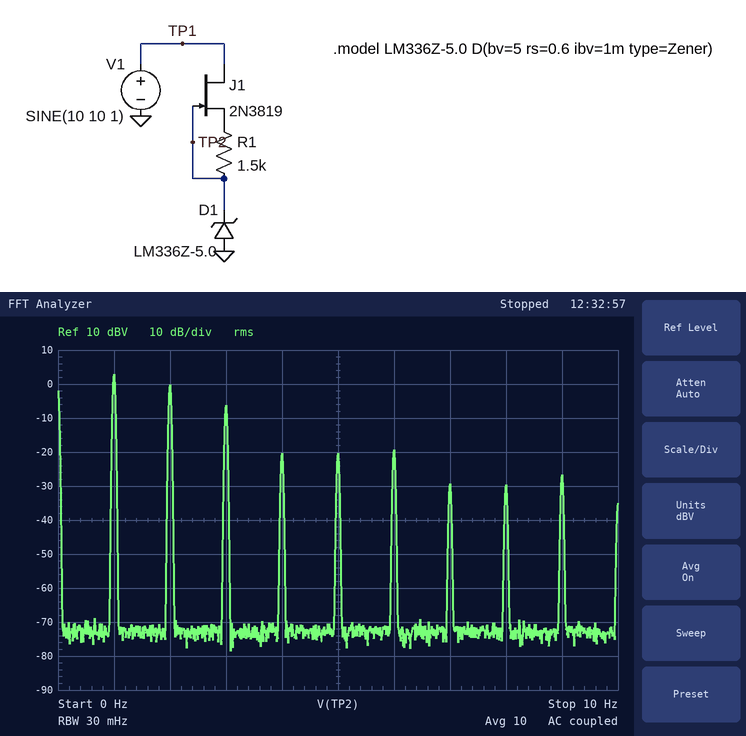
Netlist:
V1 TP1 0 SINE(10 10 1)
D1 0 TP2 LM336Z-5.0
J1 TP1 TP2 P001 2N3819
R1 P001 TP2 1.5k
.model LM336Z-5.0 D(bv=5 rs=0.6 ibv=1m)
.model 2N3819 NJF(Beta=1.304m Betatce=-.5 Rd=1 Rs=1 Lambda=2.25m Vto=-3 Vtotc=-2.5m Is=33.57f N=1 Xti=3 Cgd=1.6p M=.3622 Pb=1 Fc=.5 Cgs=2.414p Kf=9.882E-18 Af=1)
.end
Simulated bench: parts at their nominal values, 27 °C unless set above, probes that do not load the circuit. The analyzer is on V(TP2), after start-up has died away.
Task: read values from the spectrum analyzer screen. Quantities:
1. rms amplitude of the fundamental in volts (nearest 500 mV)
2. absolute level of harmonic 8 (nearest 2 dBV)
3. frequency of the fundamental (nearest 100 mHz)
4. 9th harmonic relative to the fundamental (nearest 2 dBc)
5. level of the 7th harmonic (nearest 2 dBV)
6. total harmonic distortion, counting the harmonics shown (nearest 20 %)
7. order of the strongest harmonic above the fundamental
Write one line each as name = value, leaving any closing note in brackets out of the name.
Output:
rms amplitude of the fundamental in volts = 1.5 V
absolute level of harmonic 8 = -30 dBV
frequency of the fundamental = 1.0 Hz
9th harmonic relative to the fundamental = -30 dBc
level of the 7th harmonic = -30 dBV
total harmonic distortion, counting the harmonics shown = 80 %
order of the strongest harmonic above the fundamental = 2
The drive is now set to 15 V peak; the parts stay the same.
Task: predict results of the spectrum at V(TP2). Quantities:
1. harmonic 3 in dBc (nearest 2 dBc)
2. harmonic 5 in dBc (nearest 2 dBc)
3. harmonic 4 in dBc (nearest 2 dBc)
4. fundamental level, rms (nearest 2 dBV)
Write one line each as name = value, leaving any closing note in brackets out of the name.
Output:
harmonic 3 in dBc = -20 dBc
harmonic 5 in dBc = -18 dBc
harmonic 4 in dBc = -18 dBc
fundamental level, rms = 8 dBV
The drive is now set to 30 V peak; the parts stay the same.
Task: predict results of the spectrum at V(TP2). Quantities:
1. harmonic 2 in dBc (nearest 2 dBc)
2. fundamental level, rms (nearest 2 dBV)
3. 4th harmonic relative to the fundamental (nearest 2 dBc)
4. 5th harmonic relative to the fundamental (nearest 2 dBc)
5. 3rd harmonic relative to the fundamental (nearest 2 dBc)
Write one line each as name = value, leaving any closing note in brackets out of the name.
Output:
harmonic 2 in dBc = -8 dBc
fundamental level, rms = 14 dBV
4th harmonic relative to the fundamental = -18 dBc
5th harmonic relative to the fundamental = -36 dBc
3rd harmonic relative to the fundamental = -34 dBc
